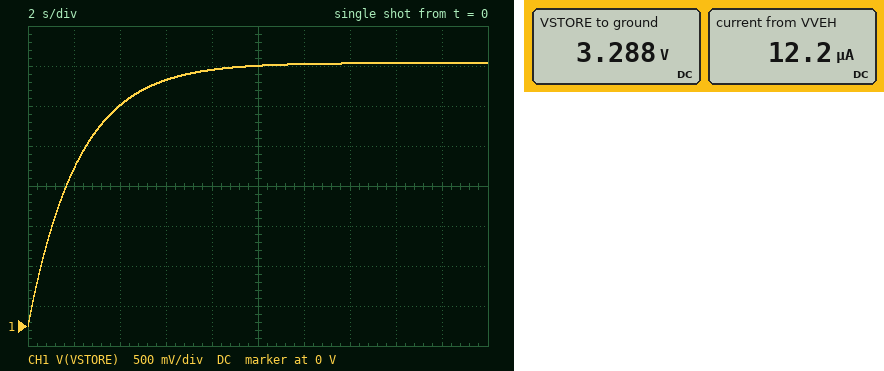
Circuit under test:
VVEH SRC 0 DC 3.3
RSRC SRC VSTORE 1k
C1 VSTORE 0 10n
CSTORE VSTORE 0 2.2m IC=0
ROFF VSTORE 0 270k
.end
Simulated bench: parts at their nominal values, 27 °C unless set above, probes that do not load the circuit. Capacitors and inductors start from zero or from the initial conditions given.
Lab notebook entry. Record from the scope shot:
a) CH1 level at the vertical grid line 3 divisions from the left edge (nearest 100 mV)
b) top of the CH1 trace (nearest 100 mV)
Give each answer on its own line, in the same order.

3.1 V
3.3 V
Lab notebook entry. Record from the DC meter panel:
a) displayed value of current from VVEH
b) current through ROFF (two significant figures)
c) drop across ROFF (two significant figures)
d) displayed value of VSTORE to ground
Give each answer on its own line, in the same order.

12.2 µA
12 µA
3.3 V
3.288 V
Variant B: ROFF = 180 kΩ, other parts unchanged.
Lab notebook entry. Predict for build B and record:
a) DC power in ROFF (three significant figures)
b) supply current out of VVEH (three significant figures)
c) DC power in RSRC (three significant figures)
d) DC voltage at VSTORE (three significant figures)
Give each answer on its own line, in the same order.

59.8 µW
18.2 µA
332 nW
3.28 V
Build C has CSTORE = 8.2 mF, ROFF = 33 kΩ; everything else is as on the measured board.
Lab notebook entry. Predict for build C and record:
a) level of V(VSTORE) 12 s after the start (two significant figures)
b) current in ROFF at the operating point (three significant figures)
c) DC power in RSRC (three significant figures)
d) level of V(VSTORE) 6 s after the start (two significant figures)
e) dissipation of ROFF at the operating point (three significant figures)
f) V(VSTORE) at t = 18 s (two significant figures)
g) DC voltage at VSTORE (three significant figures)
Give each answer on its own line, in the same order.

2.5 V
97.1 µA
9.42 µW
1.7 V
311 µW
2.9 V
3.20 V
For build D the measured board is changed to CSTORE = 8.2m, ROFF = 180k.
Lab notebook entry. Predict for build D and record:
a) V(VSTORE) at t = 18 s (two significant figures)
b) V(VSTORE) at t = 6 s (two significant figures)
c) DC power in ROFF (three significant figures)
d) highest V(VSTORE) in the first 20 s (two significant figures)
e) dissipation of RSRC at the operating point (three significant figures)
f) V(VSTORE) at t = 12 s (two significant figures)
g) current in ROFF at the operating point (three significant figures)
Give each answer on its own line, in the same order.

2.9 V
1.7 V
59.8 µW
3.0 V
332 nW
2.5 V
18.2 µA
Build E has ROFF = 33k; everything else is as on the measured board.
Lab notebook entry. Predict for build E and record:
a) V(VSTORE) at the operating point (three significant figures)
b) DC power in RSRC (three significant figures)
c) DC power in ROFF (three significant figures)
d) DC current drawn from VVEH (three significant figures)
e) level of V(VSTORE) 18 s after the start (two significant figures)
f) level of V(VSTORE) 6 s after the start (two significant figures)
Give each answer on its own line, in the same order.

3.20 V
9.42 µW
311 µW
97.1 µA
3.2 V
3.0 V
